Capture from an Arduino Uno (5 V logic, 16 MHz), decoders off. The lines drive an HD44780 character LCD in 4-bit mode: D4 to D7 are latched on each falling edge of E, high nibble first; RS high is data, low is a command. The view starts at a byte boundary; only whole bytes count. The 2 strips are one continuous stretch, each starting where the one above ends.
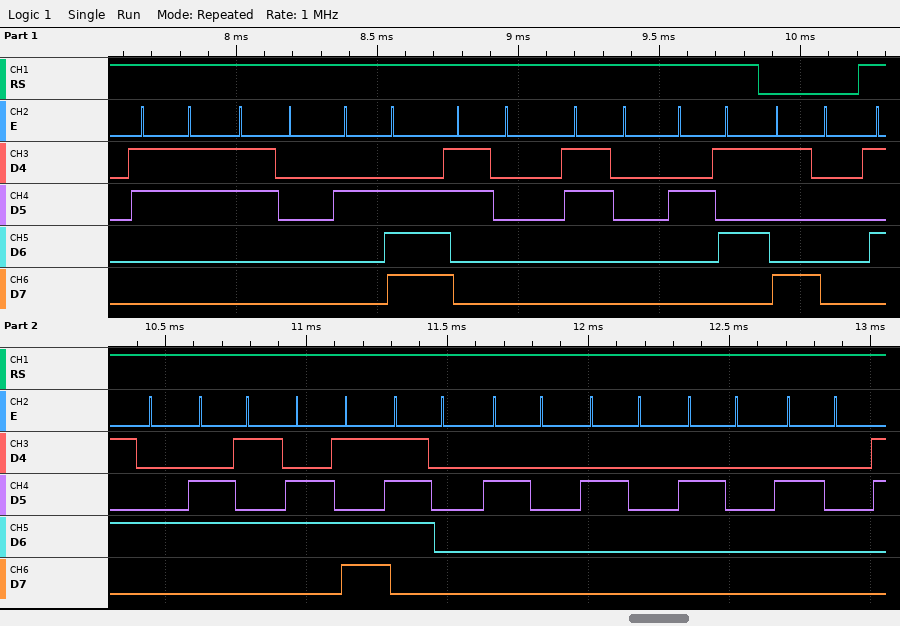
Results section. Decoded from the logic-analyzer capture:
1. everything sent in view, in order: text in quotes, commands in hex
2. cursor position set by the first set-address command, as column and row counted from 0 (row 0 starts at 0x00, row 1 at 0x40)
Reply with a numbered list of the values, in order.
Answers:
1. "30.00%" 0x90 "Temp    "
2. column 16, row 0
